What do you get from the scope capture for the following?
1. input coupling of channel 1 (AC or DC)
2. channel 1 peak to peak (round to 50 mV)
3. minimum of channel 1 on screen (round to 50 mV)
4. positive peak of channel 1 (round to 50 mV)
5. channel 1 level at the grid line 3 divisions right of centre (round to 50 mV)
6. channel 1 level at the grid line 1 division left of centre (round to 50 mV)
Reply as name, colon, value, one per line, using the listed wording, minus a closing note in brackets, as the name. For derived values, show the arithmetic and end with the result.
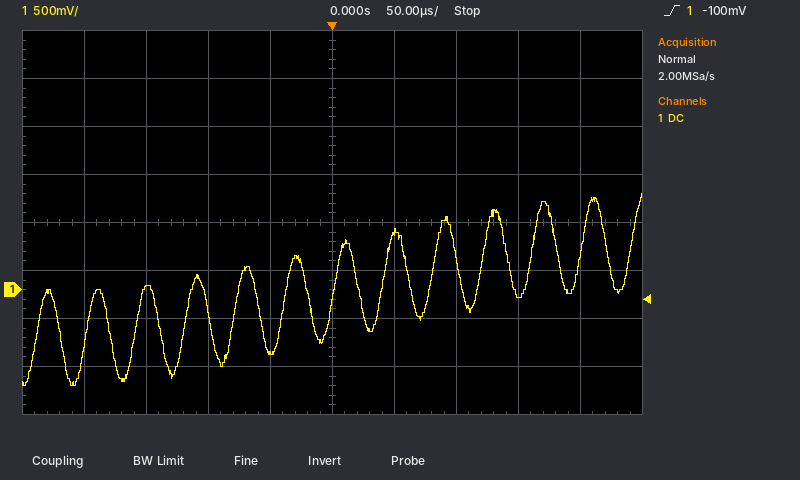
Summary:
input coupling of channel 1: DC
channel 1 peak to peak: 1.00 V − (-1.00 V) = 2.00 V
minimum of channel 1 on screen: -1.00 V
positive peak of channel 1: 1.00 V
channel 1 level at the grid line 3 divisions right of centre: -50 mV
channel 1 level at the grid line 1 division left of centre: -650 mV
